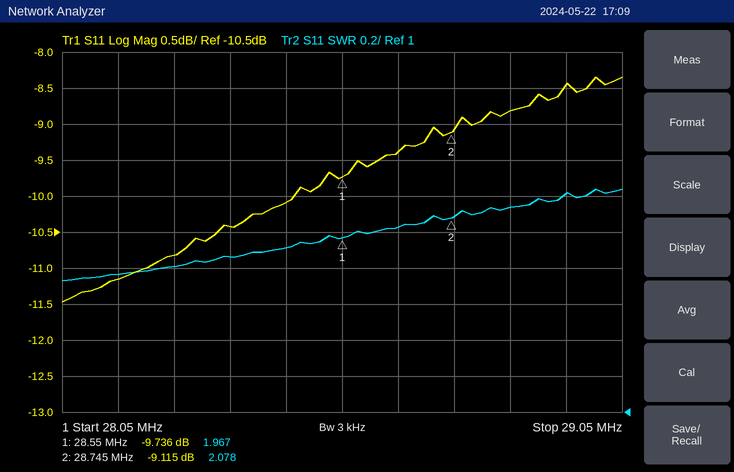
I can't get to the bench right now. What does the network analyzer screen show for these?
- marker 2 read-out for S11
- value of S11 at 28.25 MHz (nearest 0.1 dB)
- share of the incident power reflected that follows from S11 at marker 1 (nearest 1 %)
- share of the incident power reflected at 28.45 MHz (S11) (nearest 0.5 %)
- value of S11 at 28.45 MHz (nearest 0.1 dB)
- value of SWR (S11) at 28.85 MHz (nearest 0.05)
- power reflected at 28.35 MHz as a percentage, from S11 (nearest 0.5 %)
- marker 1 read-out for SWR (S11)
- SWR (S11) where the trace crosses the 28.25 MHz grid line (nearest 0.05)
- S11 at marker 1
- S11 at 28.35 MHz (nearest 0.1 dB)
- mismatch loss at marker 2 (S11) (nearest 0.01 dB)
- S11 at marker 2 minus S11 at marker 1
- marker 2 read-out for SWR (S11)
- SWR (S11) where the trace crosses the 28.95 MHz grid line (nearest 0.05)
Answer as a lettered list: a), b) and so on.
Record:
a) -9.115 dB
b) -10.8 dB
c) 11 %
d) 10.0 %
e) -10.1 dB
f) 2.15
g) 9.0 %
h) 1.967
i) 1.80
j) -9.736 dB
k) -10.4 dB
l) 0.57 dB
m) 0.621 dB
n) 2.078
o) 2.20
